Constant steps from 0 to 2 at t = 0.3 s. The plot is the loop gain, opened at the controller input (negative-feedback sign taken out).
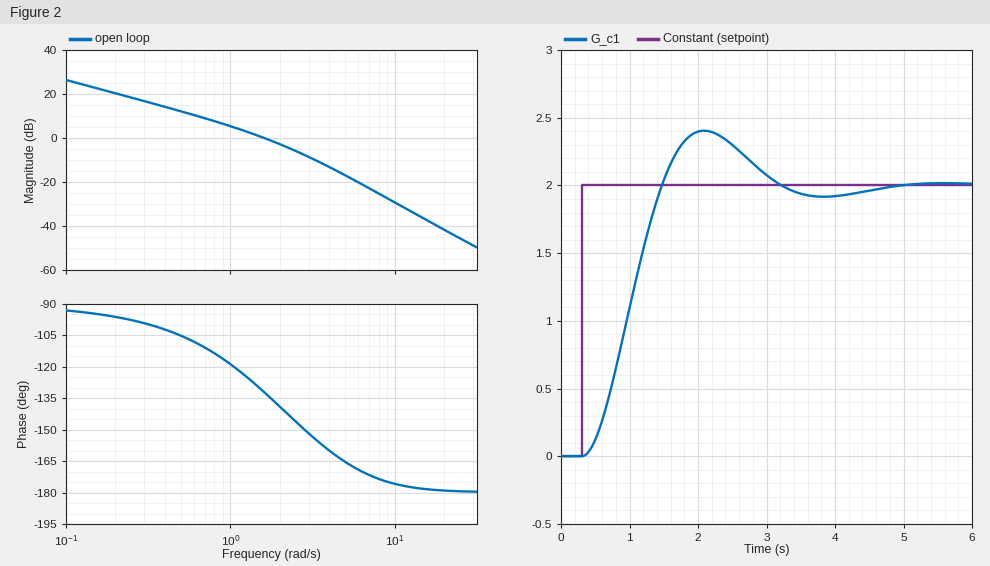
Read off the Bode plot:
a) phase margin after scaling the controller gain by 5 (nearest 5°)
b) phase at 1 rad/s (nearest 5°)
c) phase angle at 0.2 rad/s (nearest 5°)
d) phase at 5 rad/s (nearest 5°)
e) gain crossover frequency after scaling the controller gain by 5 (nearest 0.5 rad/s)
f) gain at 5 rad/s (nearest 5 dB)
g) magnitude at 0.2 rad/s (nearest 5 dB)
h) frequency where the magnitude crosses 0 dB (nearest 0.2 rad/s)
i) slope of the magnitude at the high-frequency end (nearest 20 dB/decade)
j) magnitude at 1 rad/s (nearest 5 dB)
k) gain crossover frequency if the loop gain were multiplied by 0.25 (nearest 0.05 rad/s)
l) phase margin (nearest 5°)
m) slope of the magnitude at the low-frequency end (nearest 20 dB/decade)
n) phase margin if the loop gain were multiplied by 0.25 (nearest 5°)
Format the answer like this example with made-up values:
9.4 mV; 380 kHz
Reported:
20°; -120°; -95°; -165°; 4.0 rad/s; -15 dB; 20 dB; 1.6 rad/s; -40 dB/decade; 5 dB; 0.50 rad/s; 50°; -20 dB/decade; 75°
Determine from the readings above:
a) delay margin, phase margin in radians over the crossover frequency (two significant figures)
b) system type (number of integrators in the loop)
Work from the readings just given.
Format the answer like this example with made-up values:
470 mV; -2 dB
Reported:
0.55 s; 1
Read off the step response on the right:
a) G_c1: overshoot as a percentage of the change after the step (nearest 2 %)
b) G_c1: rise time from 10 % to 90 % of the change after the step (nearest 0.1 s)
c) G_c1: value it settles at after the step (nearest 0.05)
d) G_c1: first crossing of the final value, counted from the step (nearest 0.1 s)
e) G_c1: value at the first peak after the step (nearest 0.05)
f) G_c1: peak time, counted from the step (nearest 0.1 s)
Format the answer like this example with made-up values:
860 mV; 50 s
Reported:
20 %; 0.8 s; 2.00; 1.2 s; 2.40; 1.8 s
